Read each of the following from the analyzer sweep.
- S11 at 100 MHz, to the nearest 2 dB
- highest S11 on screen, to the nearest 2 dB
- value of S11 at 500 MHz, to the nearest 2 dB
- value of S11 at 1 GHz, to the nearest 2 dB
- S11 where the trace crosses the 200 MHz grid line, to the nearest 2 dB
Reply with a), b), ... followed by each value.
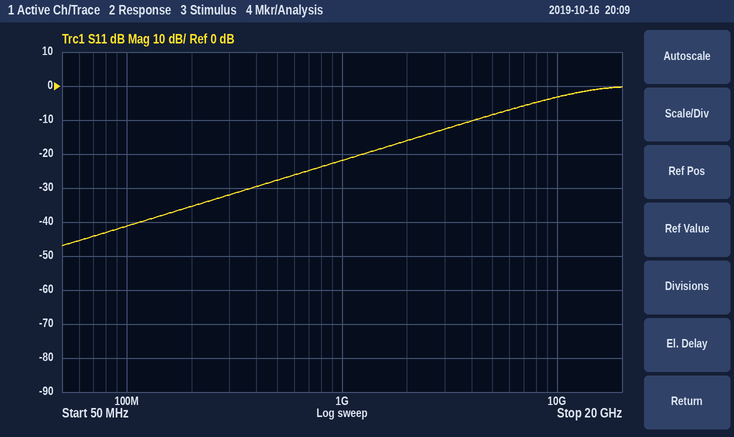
a) -42 dB
b) 0 dB
c) -28 dB
d) -22 dB
e) -36 dB
